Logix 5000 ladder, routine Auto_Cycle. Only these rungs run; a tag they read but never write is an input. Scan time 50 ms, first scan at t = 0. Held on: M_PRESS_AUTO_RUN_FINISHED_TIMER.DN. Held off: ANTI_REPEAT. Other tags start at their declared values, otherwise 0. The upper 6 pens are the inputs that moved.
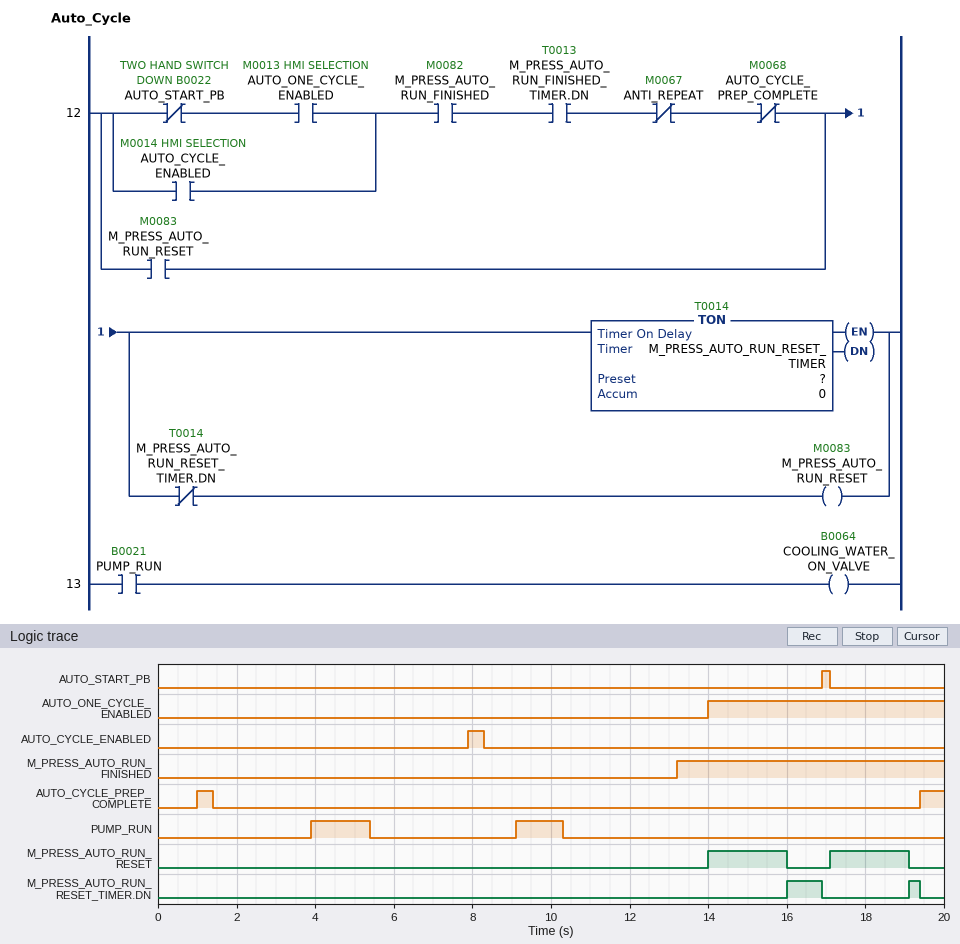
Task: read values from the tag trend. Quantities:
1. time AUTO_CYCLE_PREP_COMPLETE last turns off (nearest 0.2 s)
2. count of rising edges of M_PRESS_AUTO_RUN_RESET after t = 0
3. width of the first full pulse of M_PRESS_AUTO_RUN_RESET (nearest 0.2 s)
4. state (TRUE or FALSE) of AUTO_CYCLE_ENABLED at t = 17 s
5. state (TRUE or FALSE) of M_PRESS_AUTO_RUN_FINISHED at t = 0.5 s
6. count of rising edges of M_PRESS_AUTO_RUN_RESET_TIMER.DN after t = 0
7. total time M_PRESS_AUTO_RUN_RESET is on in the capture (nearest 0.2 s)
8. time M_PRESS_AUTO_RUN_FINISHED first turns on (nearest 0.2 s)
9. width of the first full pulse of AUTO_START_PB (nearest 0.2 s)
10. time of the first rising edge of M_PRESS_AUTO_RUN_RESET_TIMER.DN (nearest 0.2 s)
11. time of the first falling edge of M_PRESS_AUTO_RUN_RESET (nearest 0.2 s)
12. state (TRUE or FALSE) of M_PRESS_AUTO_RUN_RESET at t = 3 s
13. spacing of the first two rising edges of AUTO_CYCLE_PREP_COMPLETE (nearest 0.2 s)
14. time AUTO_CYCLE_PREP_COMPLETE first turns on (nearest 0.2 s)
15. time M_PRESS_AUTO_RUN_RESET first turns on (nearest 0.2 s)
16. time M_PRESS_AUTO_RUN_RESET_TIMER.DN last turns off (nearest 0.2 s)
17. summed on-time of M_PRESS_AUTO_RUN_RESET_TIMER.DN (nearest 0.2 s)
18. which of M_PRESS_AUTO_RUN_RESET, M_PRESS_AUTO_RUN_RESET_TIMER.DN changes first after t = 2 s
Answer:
1.4 s
2
2.0 s
FALSE
FALSE
2
4.0 s
13.2 s
0.2 s
16.0 s
16.0 s
FALSE
18.4 s
1.0 s
14.0 s
19.4 s
1.2 s
M_PRESS_AUTO_RUN_RESET
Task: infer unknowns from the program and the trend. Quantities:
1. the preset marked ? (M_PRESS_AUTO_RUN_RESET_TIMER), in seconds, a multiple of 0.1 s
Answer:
2.0 s
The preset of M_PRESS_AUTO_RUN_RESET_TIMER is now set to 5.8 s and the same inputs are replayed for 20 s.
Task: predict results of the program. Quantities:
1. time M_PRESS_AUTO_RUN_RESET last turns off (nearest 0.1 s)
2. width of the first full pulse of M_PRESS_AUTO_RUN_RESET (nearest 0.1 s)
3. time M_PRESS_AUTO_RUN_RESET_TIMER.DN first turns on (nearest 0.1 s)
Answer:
19.8 s
5.8 s
19.8 s
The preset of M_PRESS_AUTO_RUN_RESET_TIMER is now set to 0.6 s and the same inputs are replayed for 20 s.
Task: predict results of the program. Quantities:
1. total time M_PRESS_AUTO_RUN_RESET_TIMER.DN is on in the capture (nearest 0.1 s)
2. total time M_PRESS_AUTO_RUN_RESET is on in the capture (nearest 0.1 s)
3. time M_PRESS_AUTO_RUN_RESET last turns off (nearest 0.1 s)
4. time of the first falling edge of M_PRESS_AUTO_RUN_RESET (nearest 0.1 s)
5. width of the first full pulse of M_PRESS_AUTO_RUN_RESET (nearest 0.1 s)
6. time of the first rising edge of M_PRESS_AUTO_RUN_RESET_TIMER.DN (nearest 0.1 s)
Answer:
4.0 s
1.2 s
17.7 s
14.6 s
0.6 s
14.6 s
